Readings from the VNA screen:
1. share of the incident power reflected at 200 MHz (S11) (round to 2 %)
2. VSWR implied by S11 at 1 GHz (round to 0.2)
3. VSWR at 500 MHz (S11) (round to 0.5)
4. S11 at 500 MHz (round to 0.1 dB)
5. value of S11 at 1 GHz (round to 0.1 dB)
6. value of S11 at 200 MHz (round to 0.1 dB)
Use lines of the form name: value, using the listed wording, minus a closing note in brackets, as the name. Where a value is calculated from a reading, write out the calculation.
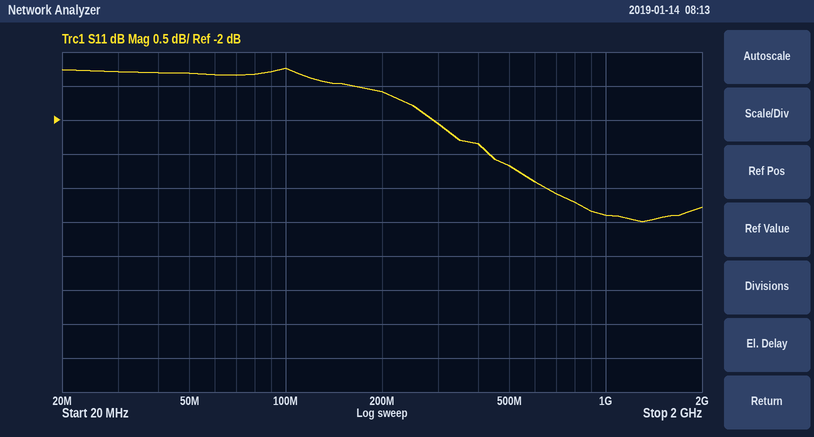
share of the incident power reflected at 200 MHz (S11): 10^(-1.6/10) ≈ 69.2 %, so 70 % to the nearest 2 %
VSWR implied by S11 at 1 GHz: |Γ| = 10^(-3.4/20) = 0.6761; VSWR = (1 + 0.6761)/(1 − 0.6761) ≈ 5.2
VSWR at 500 MHz (S11): |Γ| = 10^(-2.7/20) = 0.7328; VSWR = (1 + 0.7328)/(1 − 0.7328) ≈ 6.5
S11 at 500 MHz: -2.7 dB
value of S11 at 1 GHz: -3.4 dB
value of S11 at 200 MHz: -1.6 dB
